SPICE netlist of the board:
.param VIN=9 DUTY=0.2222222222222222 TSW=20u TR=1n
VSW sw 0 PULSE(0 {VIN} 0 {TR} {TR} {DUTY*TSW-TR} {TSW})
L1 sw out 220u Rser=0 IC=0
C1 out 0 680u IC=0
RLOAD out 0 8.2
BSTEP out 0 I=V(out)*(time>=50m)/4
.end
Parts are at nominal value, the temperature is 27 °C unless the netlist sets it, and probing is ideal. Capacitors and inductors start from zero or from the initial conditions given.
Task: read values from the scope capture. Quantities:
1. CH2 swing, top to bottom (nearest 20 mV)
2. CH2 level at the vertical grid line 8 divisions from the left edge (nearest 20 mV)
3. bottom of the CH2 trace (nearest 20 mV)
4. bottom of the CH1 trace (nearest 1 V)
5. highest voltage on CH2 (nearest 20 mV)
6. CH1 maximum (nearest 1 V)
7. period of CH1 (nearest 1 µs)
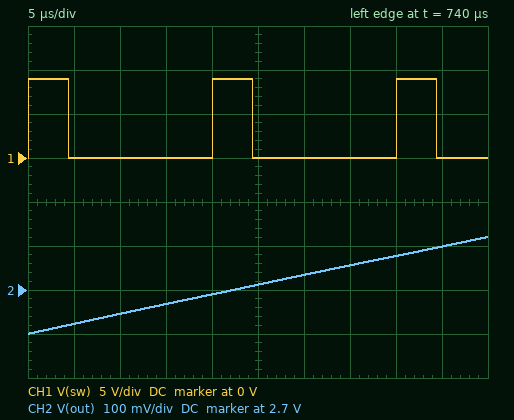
220 mV
2.78 V
2.60 V
0 V
2.82 V
9 V
20 µs
